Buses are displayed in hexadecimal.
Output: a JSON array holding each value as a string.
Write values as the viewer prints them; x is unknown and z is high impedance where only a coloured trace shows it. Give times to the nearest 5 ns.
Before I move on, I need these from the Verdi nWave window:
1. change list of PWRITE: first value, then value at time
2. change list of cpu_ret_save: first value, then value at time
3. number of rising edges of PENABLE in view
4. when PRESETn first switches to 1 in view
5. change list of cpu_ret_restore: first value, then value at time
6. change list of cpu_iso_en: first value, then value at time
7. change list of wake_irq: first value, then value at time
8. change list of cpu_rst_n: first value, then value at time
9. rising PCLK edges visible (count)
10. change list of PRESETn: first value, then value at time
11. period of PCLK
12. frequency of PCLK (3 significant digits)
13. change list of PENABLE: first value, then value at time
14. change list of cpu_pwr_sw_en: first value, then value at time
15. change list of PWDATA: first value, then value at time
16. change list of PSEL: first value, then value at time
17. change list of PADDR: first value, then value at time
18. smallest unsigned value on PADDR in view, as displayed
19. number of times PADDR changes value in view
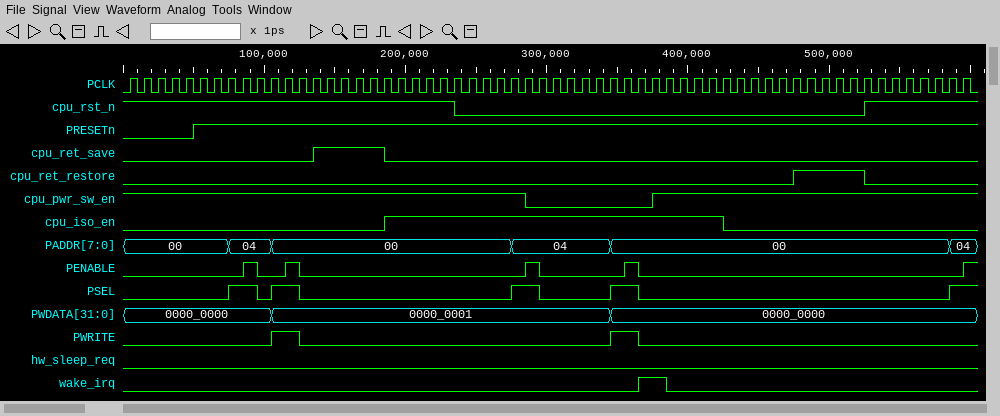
["0, 1 at 105 ns, 0 at 125 ns, 1 at 345 ns, 0 at 365 ns", "0, 1 at 135 ns, 0 at 185 ns", "5", "50 ns", "0, 1 at 475 ns, 0 at 525 ns", "0, 1 at 185 ns, 0 at 425 ns", "0, 1 at 365 ns, 0 at 385 ns", "1, 0 at 235 ns, 1 at 525 ns", "60", "0, 1 at 50 ns", "10 ns", "100 MHz", "0, 1 at 85 ns, 0 at 95 ns, 1 at 115 ns, 0 at 125 ns, 1 at 285 ns, 0 at 295 ns, 1 at 355 ns, 0 at 365 ns, 1 at 595 ns", "1, 0 at 285 ns, 1 at 375 ns", "0000_0000, 0000_0001 at 105 ns, 0000_0000 at 345 ns", "0, 1 at 75 ns, 0 at 95 ns, 1 at 105 ns, 0 at 125 ns, 1 at 275 ns, 0 at 295 ns, 1 at 345 ns, 0 at 365 ns, 1 at 585 ns", "00, 04 at 75 ns, 00 at 105 ns, 04 at 275 ns, 00 at 345 ns, 04 at 585 ns", "00", "5"]
